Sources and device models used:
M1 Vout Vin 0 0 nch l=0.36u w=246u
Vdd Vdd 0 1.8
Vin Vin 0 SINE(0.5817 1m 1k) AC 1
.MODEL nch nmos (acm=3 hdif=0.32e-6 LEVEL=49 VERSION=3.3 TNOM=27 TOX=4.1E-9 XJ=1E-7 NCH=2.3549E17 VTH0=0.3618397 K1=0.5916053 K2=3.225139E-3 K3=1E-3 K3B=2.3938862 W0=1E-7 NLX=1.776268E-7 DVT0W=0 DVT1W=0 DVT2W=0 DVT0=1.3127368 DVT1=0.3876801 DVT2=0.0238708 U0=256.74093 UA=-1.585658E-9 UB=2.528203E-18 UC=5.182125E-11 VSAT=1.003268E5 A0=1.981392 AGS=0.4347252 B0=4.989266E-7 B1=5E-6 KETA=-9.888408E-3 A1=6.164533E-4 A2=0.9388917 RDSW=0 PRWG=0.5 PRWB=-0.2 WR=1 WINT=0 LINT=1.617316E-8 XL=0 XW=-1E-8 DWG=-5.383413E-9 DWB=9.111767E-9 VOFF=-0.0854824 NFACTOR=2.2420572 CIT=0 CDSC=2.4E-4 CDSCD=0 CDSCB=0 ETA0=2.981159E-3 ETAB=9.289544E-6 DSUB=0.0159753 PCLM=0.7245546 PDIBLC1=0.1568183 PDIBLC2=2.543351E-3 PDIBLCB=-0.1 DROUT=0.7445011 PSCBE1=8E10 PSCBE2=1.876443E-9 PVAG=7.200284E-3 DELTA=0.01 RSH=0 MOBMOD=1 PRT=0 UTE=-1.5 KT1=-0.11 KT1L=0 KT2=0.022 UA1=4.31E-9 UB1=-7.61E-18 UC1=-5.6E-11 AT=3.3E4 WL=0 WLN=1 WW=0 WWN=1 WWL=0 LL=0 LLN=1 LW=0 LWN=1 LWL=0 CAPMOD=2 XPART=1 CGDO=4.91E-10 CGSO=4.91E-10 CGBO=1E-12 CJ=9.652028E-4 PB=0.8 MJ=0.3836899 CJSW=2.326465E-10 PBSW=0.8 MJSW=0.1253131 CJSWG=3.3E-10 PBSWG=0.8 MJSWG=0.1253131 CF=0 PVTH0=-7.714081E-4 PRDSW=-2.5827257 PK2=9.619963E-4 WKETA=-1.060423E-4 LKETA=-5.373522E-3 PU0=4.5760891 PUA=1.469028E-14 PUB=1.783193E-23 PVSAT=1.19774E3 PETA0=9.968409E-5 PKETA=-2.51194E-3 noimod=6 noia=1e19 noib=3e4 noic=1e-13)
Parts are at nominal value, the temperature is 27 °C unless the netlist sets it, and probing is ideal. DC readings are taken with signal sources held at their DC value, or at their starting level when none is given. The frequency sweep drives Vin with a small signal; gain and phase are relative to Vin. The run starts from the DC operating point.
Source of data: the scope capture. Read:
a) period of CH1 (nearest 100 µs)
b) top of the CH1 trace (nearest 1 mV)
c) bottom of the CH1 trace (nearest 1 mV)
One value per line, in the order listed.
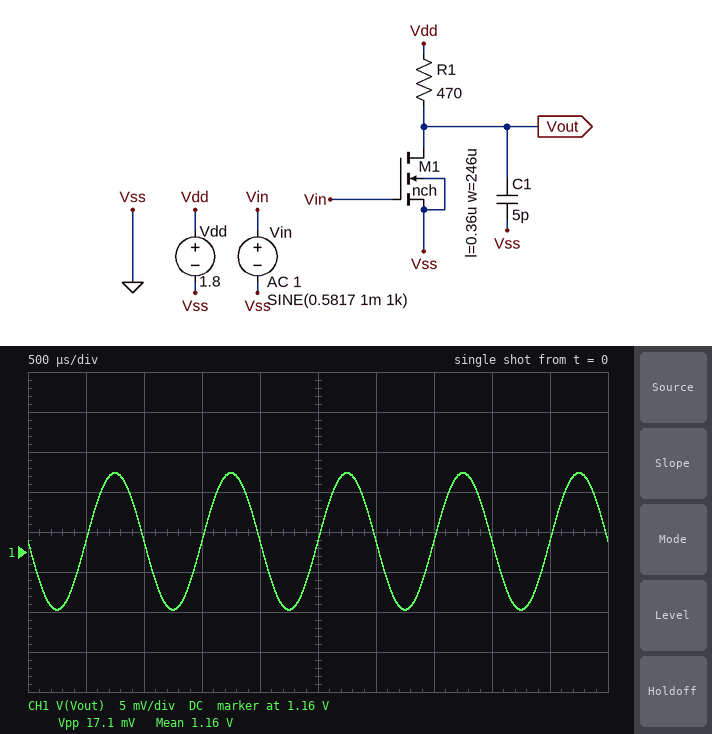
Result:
1.0 ms
1.170 V
1.153 V
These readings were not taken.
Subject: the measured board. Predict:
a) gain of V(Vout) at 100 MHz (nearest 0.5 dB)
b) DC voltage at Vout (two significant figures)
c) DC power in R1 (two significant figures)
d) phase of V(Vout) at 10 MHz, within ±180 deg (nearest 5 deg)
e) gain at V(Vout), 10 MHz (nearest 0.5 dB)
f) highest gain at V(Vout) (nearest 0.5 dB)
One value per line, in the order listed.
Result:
14.0 dB
1.2 V
870 µW
170 deg
18.5 dB
18.5 dB
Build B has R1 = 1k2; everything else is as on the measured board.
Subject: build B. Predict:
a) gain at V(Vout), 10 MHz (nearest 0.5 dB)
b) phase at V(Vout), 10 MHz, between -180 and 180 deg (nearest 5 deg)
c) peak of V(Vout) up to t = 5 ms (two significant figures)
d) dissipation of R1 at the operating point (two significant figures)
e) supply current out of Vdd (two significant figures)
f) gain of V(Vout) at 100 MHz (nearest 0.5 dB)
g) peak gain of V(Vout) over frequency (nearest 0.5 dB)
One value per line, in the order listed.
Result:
24.0 dB
165 deg
400 mV
1.7 mW
1.2 mA
14.0 dB
24.5 dB
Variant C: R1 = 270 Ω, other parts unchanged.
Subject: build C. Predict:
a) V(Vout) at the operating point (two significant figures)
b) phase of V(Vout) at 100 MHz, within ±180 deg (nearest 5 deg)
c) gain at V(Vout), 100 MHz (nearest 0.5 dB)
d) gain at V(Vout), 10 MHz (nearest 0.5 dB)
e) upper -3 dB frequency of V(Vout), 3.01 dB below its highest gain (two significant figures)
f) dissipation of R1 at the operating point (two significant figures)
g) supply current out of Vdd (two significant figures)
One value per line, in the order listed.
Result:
1.4 V
140 deg
12.0 dB
14.5 dB
120 MHz
540 µW
1.4 mA
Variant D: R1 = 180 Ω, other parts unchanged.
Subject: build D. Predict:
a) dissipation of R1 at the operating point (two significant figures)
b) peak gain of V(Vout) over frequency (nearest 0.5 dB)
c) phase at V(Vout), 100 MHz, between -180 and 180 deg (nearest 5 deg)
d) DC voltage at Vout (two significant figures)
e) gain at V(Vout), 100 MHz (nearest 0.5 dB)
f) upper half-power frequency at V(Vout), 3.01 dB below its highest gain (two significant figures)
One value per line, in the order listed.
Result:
380 µW
11.0 dB
150 deg
1.5 V
10.0 dB
170 MHz
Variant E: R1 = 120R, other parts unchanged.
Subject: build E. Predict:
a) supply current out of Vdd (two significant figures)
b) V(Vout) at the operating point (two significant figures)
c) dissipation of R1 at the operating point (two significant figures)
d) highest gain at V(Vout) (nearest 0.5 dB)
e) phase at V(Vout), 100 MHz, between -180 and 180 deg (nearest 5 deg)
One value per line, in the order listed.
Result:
1.5 mA
1.6 V
260 µW
8.0 dB
160 deg
